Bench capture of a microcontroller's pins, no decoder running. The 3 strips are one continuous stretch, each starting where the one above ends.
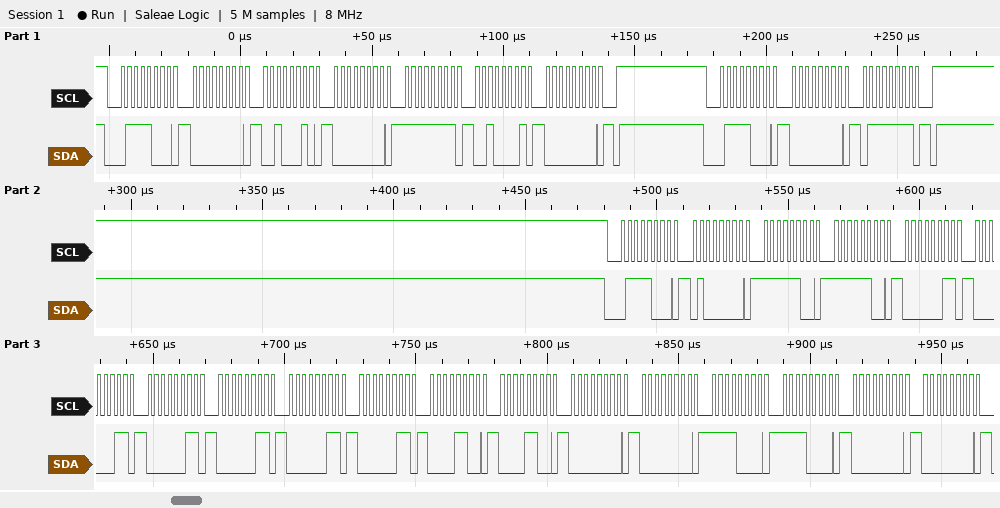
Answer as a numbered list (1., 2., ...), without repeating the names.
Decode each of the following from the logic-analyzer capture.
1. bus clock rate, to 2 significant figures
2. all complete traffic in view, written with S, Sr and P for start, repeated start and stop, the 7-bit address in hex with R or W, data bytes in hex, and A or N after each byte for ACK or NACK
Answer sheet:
1. 400 kHz
2. S 3CW A 00 A 22 A 00 A FF A 21 A 00 A P S 3CW A 00 A 7F A P S 3CW A 40 A FC A FC A 03 A 03 A 03 A 03 A 03 A 03 A 0C A 0C A 00 A 00 A F0 A F0 A 00 A 00 A
